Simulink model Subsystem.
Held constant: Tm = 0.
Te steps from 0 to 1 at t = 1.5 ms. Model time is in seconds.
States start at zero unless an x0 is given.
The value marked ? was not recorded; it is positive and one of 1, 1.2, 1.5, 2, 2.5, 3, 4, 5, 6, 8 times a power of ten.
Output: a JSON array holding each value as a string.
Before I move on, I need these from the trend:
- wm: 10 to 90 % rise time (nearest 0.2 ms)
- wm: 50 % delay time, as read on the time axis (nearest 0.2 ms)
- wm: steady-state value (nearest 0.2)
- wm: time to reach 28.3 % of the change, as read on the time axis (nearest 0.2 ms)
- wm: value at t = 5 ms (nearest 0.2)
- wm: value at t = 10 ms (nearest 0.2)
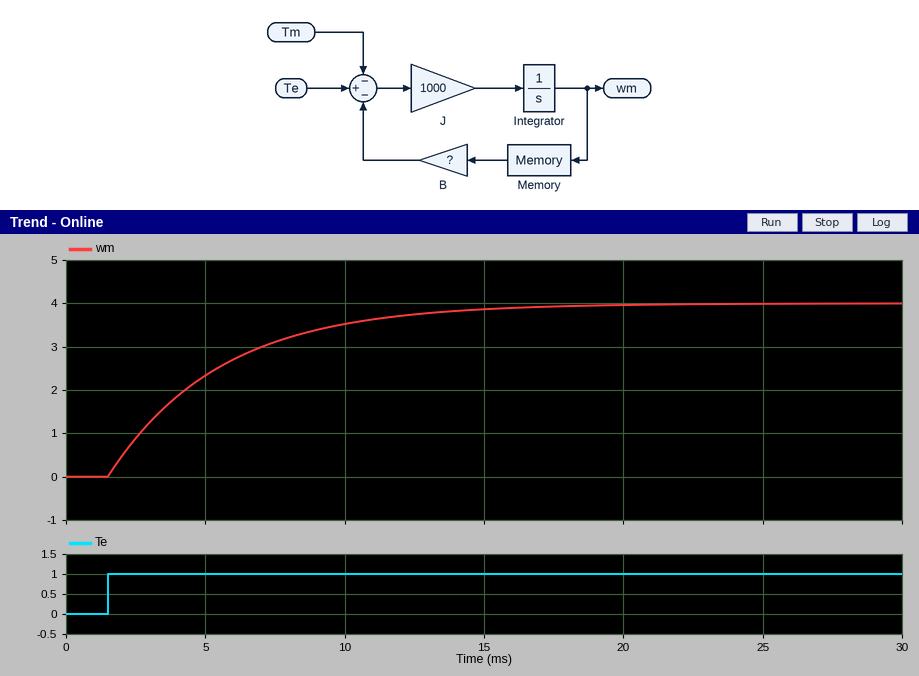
["8.8 ms", "4.2 ms", "4.0", "2.8 ms", "2.4", "3.6"]
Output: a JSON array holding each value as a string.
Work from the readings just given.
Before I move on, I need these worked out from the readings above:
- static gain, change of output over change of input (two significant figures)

["4.0"]
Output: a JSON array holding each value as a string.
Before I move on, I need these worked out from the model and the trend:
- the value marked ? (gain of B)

["0.25"]
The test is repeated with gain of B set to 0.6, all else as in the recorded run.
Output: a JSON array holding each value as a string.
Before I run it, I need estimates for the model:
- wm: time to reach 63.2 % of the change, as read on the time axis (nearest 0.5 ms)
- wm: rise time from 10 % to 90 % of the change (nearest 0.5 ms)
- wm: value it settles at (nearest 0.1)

["3.0 ms", "3.5 ms", "1.7"]
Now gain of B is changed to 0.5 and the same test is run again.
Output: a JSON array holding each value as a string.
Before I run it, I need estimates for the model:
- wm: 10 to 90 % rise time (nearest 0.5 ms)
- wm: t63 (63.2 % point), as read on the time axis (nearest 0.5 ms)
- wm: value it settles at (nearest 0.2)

["4.5 ms", "3.5 ms", "2.0"]
